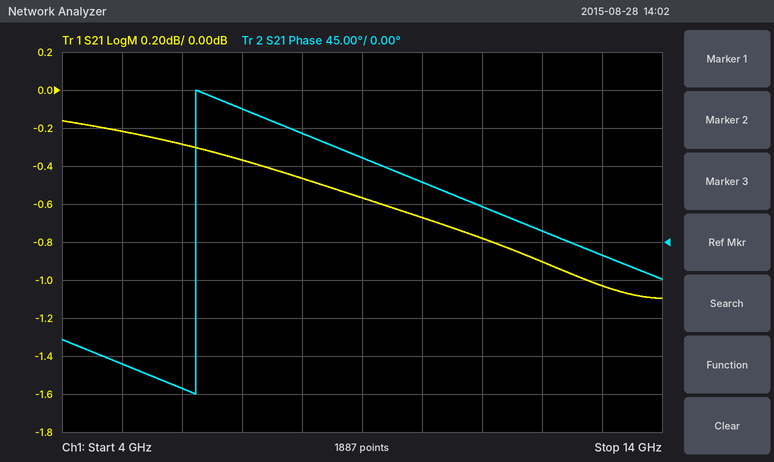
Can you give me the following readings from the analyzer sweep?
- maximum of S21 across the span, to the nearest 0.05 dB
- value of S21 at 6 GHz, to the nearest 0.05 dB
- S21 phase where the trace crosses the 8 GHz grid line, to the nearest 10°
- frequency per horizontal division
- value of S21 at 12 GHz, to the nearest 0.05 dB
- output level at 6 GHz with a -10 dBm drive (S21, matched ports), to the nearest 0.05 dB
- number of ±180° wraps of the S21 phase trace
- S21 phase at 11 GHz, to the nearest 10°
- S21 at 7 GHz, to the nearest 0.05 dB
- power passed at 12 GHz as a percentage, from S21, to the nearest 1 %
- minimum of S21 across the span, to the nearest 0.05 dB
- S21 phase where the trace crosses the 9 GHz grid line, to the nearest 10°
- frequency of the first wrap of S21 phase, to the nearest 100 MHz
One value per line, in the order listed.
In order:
-0.15 dB
-0.30 dB
130°
1 GHz
-0.90 dB
-10.30 dBm
1
40°
-0.35 dB
81 %
-1.10 dB
100°
6.2 GHz
